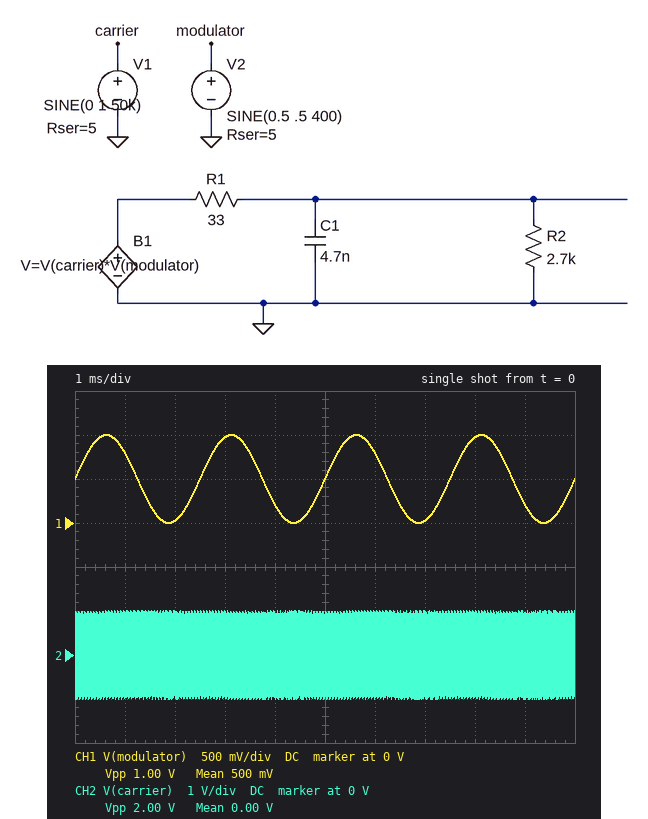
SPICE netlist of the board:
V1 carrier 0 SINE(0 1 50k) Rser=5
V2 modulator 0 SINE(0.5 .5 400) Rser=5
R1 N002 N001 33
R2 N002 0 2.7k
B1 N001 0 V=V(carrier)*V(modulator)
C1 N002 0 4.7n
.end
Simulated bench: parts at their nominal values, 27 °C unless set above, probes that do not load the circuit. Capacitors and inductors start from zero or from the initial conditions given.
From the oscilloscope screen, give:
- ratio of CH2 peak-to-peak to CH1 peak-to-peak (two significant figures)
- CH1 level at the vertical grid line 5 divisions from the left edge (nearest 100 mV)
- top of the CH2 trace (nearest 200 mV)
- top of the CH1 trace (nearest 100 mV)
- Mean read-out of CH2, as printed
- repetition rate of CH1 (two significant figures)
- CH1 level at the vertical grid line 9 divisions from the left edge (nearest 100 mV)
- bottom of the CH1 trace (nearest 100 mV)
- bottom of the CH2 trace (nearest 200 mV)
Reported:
2.0
500 mV
1.0 V
1.0 V
0.00 V
400 Hz
200 mV
0 V
-1.0 V
